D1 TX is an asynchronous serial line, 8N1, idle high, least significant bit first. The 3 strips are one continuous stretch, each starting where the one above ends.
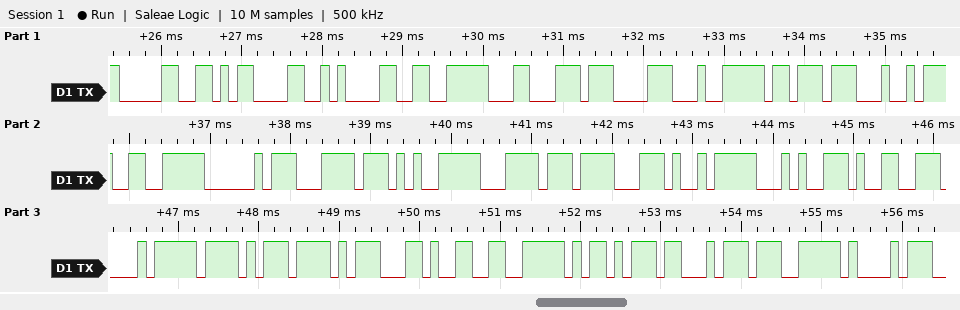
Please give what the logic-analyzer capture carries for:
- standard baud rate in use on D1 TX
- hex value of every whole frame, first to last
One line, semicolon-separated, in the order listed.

9600 baud; 30 0D 0A E6 8C 87 E4 BB A4 E6 A0 BC E5 BC 8F E9 94 99 E8 AF AF 2C E6 AD A3 E7 A1
